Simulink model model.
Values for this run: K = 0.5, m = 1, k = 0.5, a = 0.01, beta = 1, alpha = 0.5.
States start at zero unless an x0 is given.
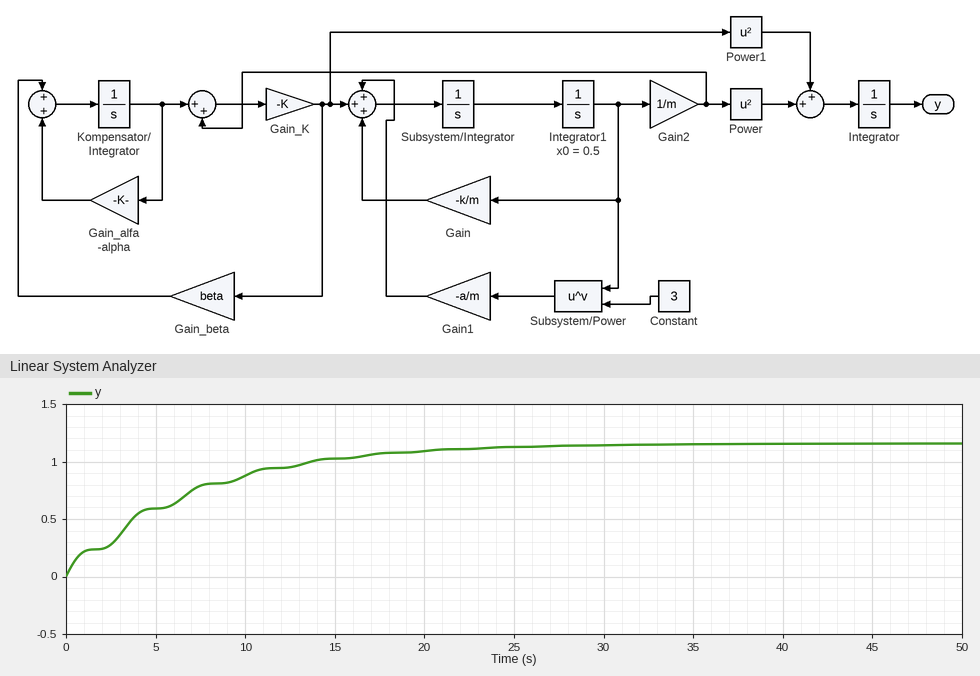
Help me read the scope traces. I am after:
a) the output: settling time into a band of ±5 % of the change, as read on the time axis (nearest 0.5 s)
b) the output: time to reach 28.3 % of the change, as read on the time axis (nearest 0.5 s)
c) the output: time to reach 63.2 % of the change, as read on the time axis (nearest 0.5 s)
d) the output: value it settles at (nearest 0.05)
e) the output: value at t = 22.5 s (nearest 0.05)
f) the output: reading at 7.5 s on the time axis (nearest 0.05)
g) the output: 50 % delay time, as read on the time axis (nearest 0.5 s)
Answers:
20.5 s
3.0 s
7.0 s
1.15
1.10
0.80
4.5 s
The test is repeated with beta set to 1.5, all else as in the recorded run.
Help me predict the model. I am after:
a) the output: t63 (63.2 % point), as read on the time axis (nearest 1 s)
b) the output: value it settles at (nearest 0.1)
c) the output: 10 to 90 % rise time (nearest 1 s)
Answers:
6 s
1.0
13 s
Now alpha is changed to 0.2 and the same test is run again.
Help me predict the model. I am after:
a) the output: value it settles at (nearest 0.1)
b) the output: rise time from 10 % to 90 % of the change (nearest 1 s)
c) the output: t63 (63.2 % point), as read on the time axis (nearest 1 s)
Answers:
0.9
11 s
5 s
